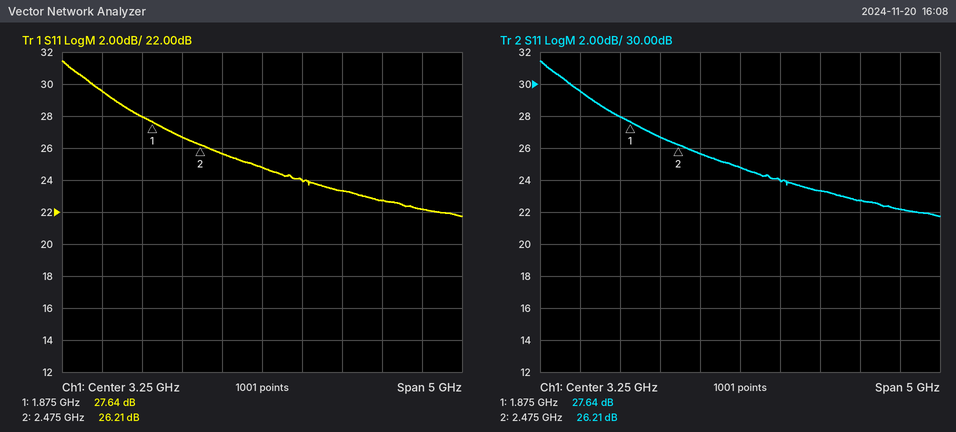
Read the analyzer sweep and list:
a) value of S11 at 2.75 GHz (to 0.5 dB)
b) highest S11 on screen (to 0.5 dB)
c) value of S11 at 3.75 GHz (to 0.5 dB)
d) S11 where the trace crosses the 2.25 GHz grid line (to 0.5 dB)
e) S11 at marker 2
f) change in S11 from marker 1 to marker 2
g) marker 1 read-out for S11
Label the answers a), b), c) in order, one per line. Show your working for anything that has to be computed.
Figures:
a) 25.5 dB
b) 31.5 dB
c) 24.0 dB
d) 26.5 dB
e) 26.21 dB
f) 26.21 − (27.64) = -1.43 dB
g) 27.64 dB
